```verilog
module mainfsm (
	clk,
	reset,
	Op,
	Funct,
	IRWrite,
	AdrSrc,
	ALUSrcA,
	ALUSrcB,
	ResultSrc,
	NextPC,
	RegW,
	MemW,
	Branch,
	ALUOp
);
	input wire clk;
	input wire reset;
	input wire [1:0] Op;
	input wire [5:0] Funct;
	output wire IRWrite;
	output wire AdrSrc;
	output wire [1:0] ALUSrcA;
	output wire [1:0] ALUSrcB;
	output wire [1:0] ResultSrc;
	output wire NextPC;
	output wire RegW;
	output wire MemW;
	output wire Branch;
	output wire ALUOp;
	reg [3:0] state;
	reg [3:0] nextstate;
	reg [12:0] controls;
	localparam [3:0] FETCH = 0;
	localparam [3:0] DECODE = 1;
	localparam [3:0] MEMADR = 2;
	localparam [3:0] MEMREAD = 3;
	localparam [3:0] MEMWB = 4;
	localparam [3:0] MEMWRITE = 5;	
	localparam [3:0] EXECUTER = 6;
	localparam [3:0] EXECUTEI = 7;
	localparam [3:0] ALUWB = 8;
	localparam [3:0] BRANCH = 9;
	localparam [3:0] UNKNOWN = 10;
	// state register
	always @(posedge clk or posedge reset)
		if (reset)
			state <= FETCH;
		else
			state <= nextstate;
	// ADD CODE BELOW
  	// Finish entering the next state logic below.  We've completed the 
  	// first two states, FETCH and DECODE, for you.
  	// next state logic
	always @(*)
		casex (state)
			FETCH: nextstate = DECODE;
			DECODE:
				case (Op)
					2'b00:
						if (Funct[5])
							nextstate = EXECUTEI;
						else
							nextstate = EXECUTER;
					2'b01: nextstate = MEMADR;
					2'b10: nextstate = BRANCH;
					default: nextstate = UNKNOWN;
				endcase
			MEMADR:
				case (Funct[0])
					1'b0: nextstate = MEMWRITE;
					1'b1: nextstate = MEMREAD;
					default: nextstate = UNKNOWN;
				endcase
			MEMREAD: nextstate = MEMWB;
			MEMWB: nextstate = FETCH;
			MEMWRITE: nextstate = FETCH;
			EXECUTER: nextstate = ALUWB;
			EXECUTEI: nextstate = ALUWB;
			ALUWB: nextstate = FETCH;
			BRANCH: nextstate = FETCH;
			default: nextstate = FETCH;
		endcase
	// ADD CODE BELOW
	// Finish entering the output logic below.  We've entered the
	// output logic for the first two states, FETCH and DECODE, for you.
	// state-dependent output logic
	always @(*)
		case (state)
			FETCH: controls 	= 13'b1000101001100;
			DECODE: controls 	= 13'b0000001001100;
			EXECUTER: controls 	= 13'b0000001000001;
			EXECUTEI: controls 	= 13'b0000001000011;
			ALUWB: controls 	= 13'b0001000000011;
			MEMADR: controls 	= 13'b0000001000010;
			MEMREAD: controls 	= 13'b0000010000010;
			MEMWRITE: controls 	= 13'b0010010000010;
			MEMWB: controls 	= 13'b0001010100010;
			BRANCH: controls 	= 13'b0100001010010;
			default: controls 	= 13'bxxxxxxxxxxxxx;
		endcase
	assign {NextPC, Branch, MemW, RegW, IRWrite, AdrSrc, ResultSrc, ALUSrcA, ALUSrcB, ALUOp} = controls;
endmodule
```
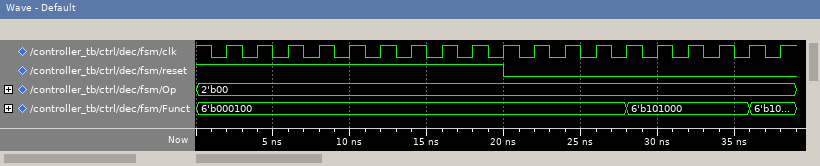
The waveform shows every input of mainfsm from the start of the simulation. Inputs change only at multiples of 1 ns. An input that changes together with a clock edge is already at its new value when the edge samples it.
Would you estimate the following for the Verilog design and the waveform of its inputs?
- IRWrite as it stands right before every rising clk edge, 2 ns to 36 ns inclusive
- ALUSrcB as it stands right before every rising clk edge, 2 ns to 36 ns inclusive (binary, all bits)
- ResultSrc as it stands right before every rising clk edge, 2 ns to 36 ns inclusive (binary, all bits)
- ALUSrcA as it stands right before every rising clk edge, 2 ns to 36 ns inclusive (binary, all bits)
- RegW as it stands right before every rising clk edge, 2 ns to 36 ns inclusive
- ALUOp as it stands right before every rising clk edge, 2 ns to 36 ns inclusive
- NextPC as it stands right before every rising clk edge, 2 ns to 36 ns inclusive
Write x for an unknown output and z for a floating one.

1 1 1 1 1 1 1 1 1 1 0 0 0 1 0 0 0 1
10, 10, 10, 10, 10, 10, 10, 10, 10, 10, 10, 00, 01, 10, 10, 01, 01, 10
10, 10, 10, 10, 10, 10, 10, 10, 10, 10, 10, 10, 00, 10, 10, 10, 00, 10
01, 01, 01, 01, 01, 01, 01, 01, 01, 01, 01, 00, 00, 01, 01, 00, 00, 01
0 0 0 0 0 0 0 0 0 0 0 0 1 0 0 0 1 0
0 0 0 0 0 0 0 0 0 0 0 1 1 0 0 1 1 0
1 1 1 1 1 1 1 1 1 1 0 0 0 1 0 0 0 1
